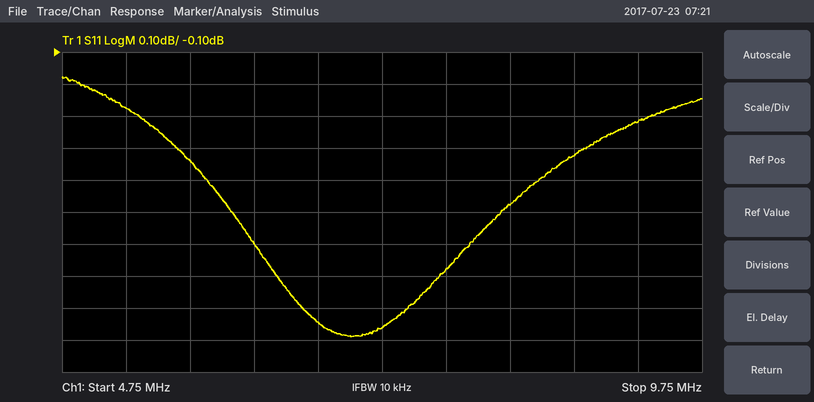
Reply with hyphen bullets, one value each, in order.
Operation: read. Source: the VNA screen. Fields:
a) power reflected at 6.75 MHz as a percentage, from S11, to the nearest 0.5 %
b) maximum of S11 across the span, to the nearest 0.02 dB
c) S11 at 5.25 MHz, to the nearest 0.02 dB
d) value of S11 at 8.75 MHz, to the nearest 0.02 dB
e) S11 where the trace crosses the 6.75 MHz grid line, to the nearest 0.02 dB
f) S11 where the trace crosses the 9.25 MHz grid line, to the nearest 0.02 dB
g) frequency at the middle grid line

- 80.5 %
- -0.18 dB
- -0.28 dB
- -0.42 dB
- -0.94 dB
- -0.32 dB
- 7.25 MHz
